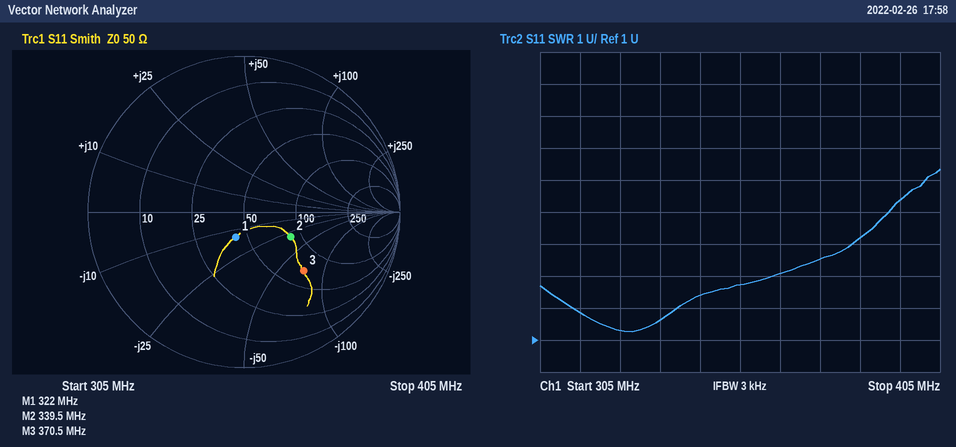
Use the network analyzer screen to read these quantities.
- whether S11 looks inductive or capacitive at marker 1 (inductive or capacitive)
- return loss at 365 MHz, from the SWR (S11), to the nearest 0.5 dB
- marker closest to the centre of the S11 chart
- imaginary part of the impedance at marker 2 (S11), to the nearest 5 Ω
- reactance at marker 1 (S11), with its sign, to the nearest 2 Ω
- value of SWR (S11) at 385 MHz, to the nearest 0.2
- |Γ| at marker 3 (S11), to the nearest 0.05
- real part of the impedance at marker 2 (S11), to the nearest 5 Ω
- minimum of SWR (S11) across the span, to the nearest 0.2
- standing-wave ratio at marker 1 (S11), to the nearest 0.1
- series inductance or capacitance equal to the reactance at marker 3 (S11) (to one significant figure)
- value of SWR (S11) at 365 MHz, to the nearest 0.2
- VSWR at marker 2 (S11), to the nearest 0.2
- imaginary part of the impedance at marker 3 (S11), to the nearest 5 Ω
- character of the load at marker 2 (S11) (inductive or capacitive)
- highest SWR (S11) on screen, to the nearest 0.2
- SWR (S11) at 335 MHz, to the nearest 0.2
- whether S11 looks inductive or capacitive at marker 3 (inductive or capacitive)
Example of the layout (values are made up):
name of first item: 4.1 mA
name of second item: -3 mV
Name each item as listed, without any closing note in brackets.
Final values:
whether S11 looks inductive or capacitive at marker 1: capacitive
return loss at 365 MHz, from the SWR (S11), to the nearest 0.5 dB: 6.0 dB
marker closest to the centre of the S11 chart: marker 1
imaginary part of the impedance at marker 2 (S11), to the nearest 5 Ω: -30 Ω
reactance at marker 1 (S11), with its sign, to the nearest 2 Ω: -14 Ω
value of SWR (S11) at 385 MHz, to the nearest 0.2: 4.2
|Γ| at marker 3 (S11), to the nearest 0.05: 0.55
real part of the impedance at marker 2 (S11), to the nearest 5 Ω: 85 Ω
minimum of SWR (S11) across the span, to the nearest 0.2: 1.2
standing-wave ratio at marker 1 (S11), to the nearest 0.1: 1.4
series inductance or capacitance equal to the reactance at marker 3 (S11): 6 pF
value of SWR (S11) at 365 MHz, to the nearest 0.2: 3.0
VSWR at marker 2 (S11), to the nearest 0.2: 2.0
imaginary part of the impedance at marker 3 (S11), to the nearest 5 Ω: -70 Ω
character of the load at marker 2 (S11): capacitive
highest SWR (S11) on screen, to the nearest 0.2: 6.4
SWR (S11) at 335 MHz, to the nearest 0.2: 1.6
whether S11 looks inductive or capacitive at marker 3: capacitive
